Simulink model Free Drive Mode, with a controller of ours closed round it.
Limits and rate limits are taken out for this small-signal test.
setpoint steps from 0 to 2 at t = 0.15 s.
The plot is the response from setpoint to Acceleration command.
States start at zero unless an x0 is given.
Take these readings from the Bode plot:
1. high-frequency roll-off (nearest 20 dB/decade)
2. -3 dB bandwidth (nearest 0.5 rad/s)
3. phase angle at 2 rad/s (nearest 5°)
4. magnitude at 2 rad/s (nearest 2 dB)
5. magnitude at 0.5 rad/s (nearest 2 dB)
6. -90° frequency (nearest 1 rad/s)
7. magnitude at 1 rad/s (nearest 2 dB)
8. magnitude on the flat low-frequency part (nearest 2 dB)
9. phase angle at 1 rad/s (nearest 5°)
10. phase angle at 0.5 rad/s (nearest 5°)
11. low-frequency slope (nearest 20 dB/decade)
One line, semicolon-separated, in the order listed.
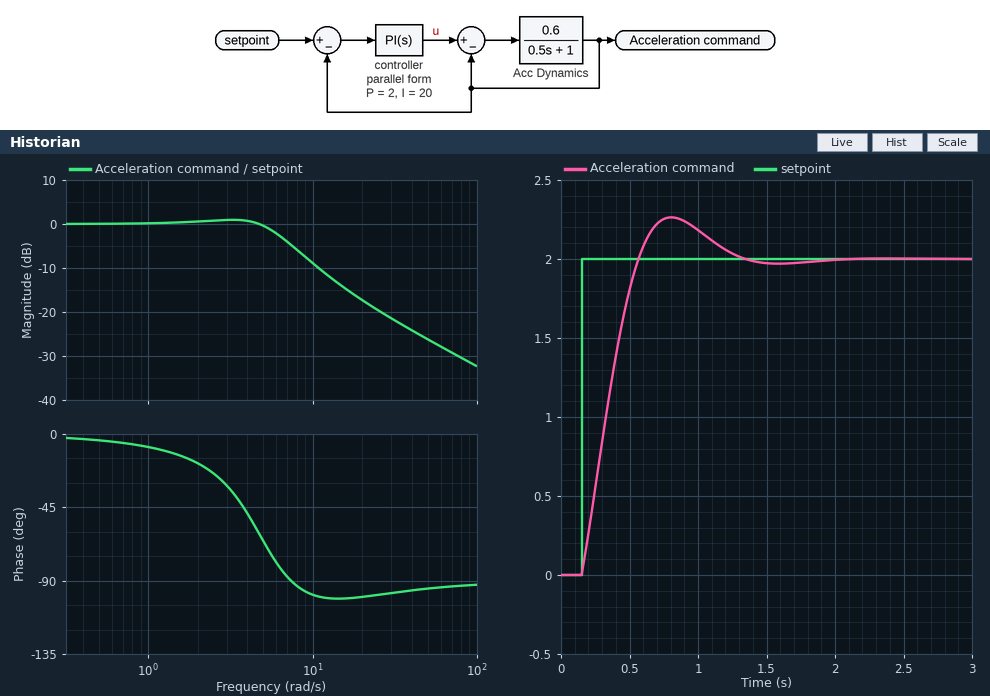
-20 dB/decade; 6.5 rad/s; -20°; 0 dB; 0 dB; 7 rad/s; 0 dB; 0 dB; -10°; -5°; 0 dB/decade
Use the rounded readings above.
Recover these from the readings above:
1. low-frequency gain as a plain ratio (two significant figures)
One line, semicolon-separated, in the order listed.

1.0
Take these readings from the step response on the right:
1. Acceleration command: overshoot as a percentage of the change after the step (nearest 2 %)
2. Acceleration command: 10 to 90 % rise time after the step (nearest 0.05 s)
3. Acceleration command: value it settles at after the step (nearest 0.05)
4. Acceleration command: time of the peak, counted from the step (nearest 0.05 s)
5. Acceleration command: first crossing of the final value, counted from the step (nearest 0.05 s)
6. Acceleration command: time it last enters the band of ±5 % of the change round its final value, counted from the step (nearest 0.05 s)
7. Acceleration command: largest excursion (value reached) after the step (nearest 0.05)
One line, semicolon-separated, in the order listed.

14 %; 0.30 s; 2.00; 0.65 s; 0.40 s; 1.00 s; 2.25
